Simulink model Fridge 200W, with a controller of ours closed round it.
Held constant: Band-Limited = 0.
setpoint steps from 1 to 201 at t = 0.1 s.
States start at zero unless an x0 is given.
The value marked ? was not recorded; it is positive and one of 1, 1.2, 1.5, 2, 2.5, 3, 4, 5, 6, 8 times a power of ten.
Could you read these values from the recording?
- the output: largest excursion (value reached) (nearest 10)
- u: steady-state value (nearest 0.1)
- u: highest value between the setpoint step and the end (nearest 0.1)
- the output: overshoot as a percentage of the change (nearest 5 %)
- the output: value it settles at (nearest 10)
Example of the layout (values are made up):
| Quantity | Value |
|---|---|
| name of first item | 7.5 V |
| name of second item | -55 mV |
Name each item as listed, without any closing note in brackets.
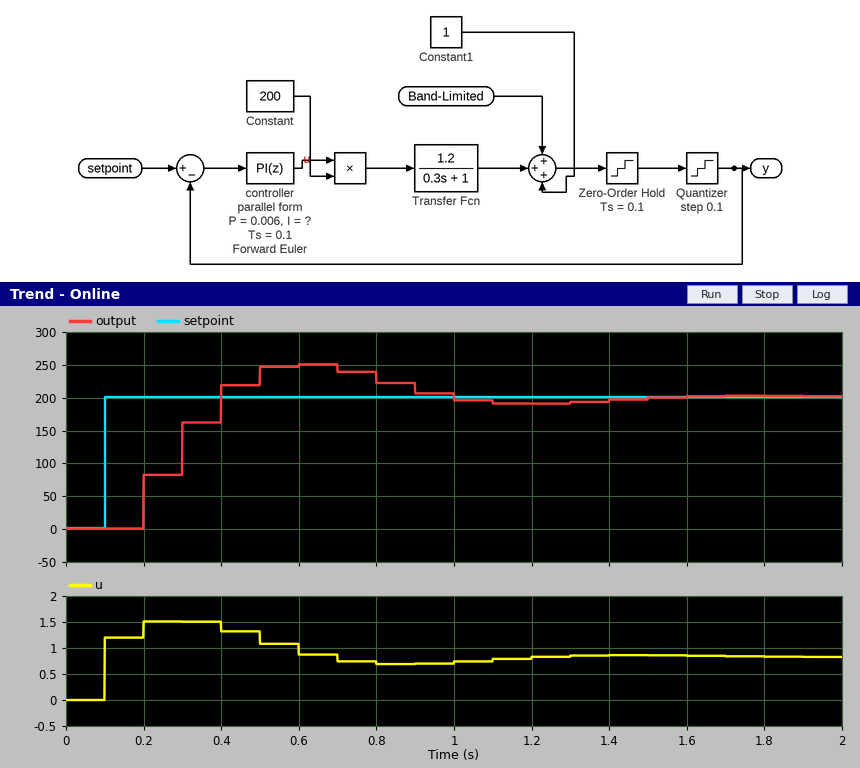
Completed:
| Quantity | Value |
|---|---|
| the output: largest excursion (value reached) | 250 |
| u: steady-state value | 0.8 |
| u: highest value between the setpoint step and the end | 1.5 |
| the output: overshoot as a percentage of the change | 25 % |
| the output: value it settles at | 200 |
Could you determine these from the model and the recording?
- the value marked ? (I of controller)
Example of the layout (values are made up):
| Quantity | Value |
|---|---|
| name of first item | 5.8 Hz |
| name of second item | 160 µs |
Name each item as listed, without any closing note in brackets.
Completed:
| Quantity | Value |
|---|---|
| the value marked ? | 0.04 |
